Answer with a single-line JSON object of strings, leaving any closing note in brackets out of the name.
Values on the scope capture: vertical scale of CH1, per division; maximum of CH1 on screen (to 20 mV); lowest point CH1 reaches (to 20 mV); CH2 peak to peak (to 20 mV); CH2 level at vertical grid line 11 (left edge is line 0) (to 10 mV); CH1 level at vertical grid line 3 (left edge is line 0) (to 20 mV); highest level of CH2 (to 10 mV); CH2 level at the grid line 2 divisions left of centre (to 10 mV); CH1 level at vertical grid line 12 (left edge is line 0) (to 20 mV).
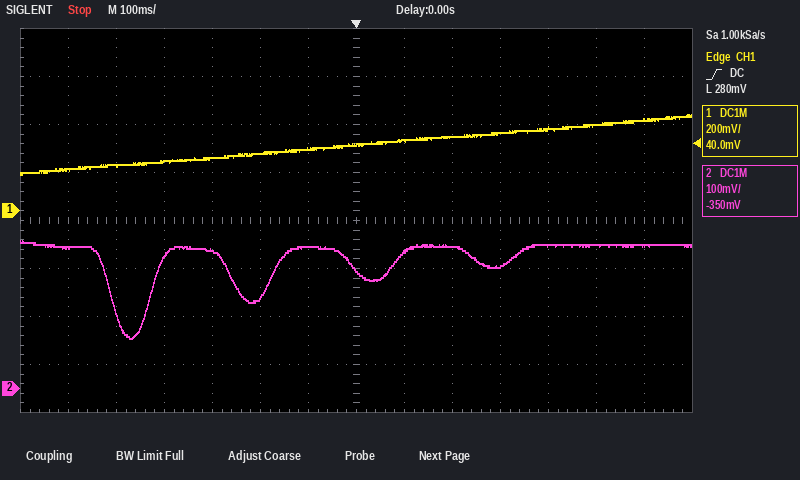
{"vertical scale of CH1, per division": "200 mV", "maximum of CH1 on screen": "400 mV", "lowest point CH1 reaches": "160 mV", "CH2 peak to peak": "200 mV", "CH2 level at vertical grid line 11 (left edge is line 0)": "300 mV", "CH1 level at vertical grid line 3 (left edge is line 0)": "200 mV", "highest level of CH2": "310 mV", "CH2 level at the grid line 2 divisions left of centre": "190 mV", "CH1 level at vertical grid line 12 (left edge is line 0)": "360 mV"}
